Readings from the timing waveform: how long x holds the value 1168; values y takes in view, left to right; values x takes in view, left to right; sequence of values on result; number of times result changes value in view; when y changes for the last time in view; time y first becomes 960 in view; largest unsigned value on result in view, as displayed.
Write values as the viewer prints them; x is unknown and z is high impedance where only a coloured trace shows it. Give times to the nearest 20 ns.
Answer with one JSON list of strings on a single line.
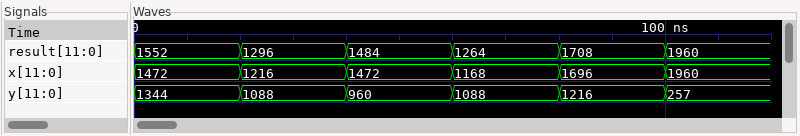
["20 ns", "1344, 1088, 960, 1088, 1216, 257", "1472, 1216, 1472, 1168, 1696, 1960", "1552, 1296, 1484, 1264, 1708, 1960", "5", "100 ns", "40 ns", "1960"]
